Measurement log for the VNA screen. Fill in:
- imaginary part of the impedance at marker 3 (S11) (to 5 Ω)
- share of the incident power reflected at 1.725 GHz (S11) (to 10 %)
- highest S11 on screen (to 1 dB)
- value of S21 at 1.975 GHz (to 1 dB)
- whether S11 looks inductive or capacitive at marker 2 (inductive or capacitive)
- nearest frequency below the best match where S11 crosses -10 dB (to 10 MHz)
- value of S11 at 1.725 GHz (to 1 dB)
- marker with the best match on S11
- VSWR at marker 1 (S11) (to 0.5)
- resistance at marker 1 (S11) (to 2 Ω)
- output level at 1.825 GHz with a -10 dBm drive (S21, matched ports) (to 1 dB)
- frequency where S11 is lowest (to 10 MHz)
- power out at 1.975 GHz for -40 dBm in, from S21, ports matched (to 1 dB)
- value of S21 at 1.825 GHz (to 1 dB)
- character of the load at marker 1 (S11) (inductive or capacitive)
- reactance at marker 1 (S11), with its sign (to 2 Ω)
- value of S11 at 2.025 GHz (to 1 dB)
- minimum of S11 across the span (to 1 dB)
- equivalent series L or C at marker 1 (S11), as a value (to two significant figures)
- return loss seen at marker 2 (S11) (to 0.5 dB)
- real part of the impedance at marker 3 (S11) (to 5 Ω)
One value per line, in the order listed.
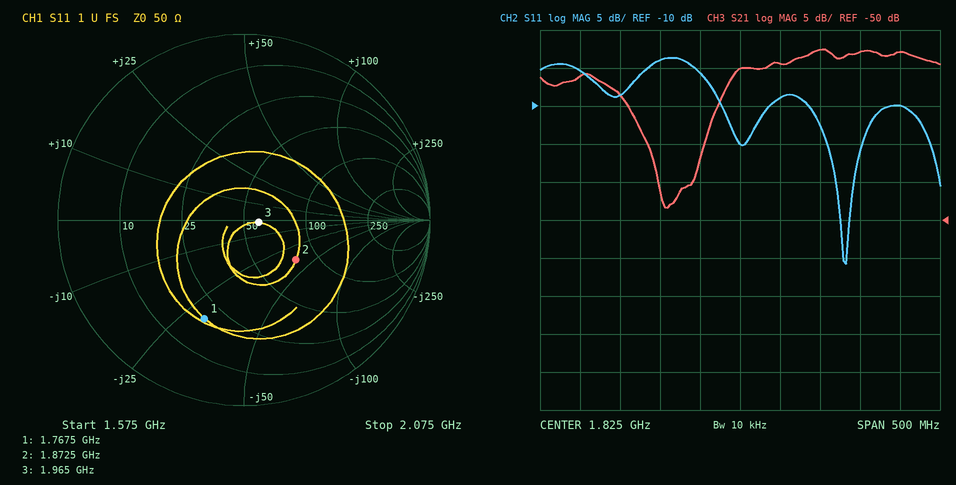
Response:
0 Ω
40 %
-4 dB
-28 dB
capacitive
1.91 GHz
-4 dB
marker 3
3.5
20 Ω
-40 dBm
1.96 GHz
-68 dBm
-30 dB
capacitive
-30 Ω
-10 dB
-31 dB
3.0 pF
9.0 dB
60 Ω
